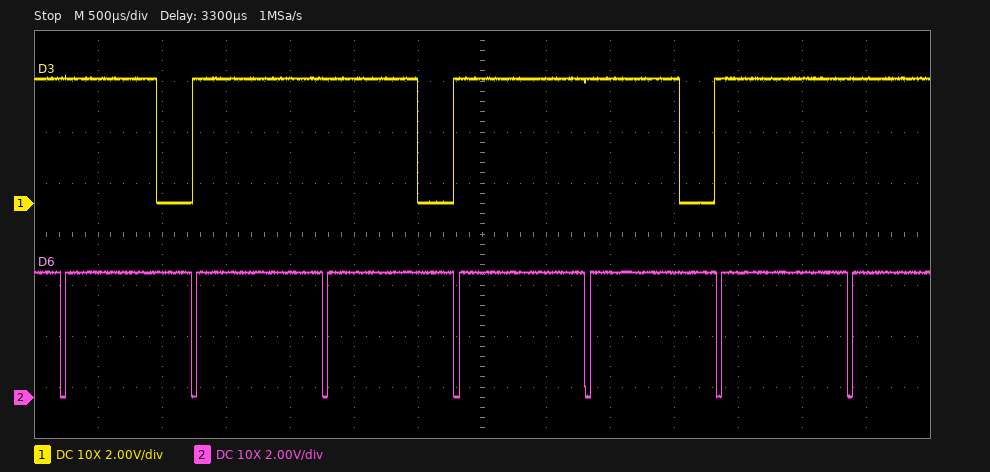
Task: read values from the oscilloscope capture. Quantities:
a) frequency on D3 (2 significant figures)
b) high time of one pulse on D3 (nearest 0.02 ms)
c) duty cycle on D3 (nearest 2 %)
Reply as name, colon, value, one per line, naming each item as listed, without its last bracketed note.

frequency on D3: 490 Hz
high time of one pulse on D3: 1.76 ms
duty cycle on D3: 86 %
